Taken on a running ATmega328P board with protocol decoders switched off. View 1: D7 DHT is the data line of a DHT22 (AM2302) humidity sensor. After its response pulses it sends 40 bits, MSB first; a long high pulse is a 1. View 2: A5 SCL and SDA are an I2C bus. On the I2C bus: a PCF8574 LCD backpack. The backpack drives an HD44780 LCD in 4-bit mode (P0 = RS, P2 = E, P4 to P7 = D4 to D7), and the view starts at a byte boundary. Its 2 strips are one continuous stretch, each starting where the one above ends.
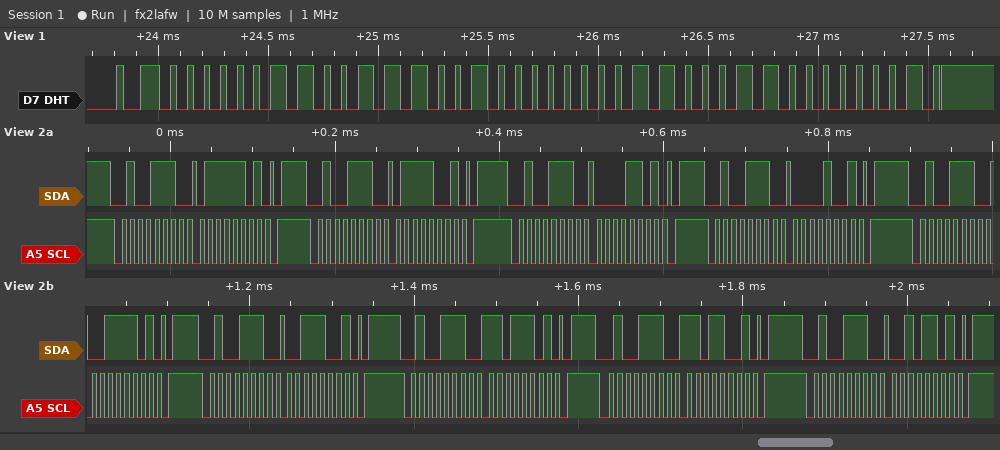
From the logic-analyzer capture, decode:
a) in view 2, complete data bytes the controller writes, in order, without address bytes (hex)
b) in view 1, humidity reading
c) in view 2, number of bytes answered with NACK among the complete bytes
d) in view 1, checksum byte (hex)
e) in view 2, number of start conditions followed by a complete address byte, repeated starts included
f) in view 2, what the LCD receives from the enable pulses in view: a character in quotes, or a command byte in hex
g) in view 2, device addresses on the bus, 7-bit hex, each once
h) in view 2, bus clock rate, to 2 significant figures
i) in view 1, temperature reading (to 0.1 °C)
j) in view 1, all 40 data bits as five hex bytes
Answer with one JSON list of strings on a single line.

["7D 79 0D 09 3D 39 DD D9 2D", "82.5 %", "0", "0x02", "9", "'p' '='", "0x27", "100 kHz", "19.8 °C", "03 39 00 C6 02"]
